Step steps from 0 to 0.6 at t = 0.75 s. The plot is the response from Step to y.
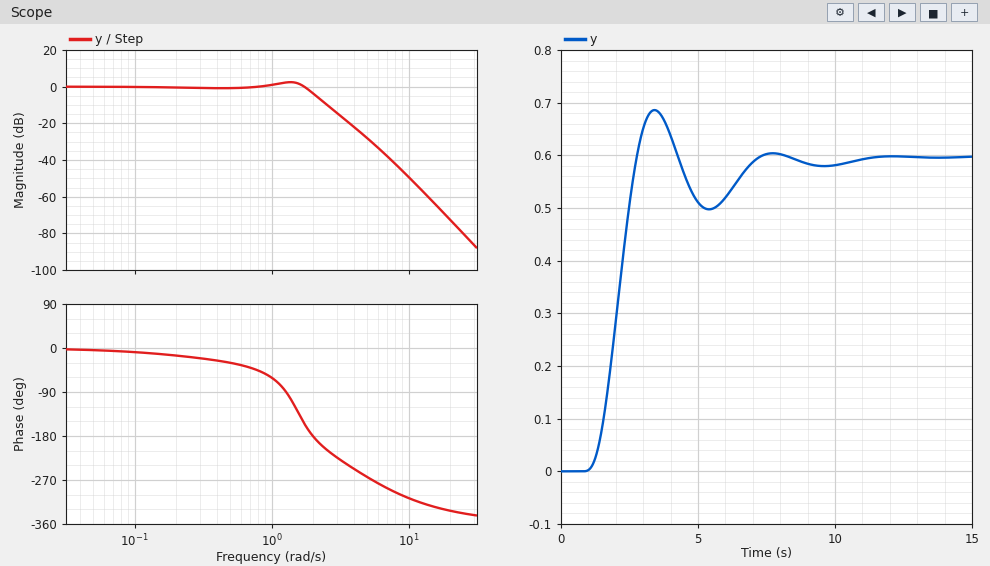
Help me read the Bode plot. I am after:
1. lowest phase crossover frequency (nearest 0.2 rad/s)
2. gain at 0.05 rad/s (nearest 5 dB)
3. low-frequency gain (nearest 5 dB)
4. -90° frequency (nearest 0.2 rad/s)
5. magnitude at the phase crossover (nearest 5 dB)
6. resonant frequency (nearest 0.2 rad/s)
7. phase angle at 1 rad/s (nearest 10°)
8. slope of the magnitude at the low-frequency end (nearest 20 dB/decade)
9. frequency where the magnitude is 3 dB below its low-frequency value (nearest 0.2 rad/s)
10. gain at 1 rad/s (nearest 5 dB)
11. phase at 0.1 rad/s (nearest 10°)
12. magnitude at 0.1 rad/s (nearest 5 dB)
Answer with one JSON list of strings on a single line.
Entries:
["2.0 rad/s", "0 dB", "0 dB", "1.2 rad/s", "-5 dB", "1.4 rad/s", "-60°", "0 dB/decade", "2.0 rad/s", "0 dB", "-10°", "0 dB"]
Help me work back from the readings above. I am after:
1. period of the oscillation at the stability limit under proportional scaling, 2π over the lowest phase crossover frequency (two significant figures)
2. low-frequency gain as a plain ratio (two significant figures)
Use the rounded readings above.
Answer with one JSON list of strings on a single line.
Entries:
["3.1 s", "1.0"]
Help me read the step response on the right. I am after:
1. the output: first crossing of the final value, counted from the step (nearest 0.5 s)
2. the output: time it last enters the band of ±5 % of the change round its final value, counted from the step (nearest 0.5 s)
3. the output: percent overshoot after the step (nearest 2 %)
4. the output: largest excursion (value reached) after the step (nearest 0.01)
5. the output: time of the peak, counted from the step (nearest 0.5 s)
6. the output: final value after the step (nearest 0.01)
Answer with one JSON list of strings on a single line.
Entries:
["2.0 s", "6.0 s", "14 %", "0.69", "2.5 s", "0.60"]
